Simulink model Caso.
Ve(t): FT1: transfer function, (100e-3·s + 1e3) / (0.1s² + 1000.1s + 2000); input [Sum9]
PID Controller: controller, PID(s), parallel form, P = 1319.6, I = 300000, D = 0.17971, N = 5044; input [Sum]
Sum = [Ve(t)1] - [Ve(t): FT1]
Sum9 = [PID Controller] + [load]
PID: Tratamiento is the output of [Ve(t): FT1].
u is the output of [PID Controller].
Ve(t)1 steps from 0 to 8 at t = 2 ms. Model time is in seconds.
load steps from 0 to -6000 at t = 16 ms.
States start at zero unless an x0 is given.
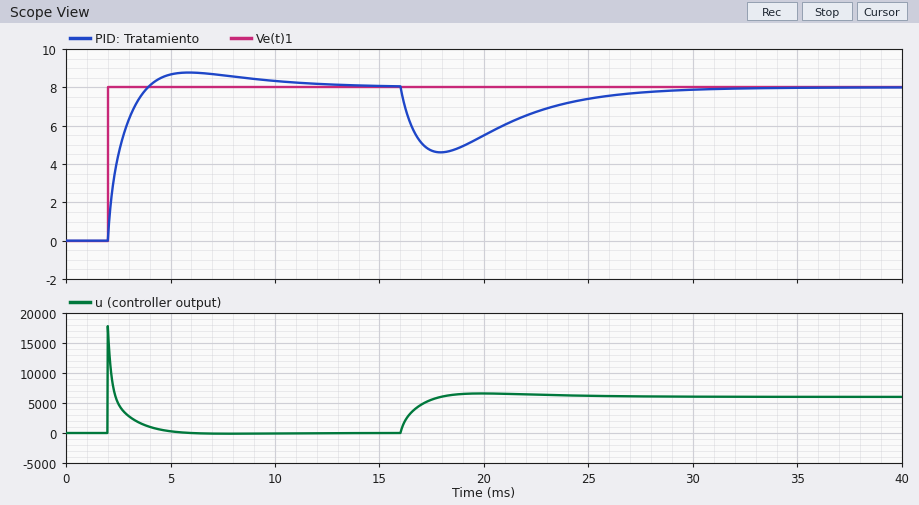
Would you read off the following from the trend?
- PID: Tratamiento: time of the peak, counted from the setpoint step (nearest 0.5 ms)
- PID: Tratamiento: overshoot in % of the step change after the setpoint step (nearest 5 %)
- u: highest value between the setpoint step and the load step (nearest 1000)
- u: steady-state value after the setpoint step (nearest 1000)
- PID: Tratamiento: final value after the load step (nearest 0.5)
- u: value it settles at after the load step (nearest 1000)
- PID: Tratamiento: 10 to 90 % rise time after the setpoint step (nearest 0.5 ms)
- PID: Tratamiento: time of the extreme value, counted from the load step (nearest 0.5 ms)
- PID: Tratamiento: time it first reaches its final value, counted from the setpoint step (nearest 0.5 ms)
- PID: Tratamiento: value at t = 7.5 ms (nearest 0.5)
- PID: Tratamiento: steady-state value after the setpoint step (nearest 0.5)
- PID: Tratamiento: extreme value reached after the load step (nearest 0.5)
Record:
4.0 ms
10 %
18000
0
8.0
6000
1.5 ms
2.0 ms
2.0 ms
8.5
8.0
4.5
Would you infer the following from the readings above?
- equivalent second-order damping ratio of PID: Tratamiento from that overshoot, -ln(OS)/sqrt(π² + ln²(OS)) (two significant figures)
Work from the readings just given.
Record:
0.59
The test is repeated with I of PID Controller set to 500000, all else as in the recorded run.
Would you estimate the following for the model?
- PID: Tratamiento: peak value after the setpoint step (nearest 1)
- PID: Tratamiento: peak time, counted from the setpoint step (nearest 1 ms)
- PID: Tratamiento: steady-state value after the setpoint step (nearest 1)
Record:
9
3 ms
8
